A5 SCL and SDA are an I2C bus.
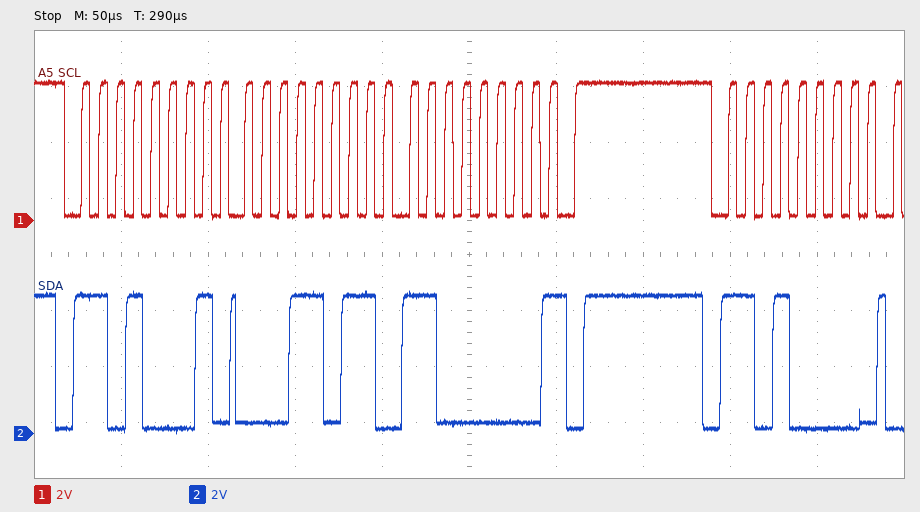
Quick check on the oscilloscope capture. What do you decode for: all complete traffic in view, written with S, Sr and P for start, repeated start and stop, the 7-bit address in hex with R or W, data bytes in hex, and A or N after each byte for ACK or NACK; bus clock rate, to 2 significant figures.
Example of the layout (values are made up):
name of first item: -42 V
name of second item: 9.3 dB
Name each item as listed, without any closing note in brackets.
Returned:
all complete traffic in view, written with S, Sr and P for start, repeated start and stop, the 7-bit address in hex with R or W, data bytes in hex, and A or N after each byte for ACK or NACK: S 68R A 1B A C0 N P S 68W A
bus clock rate, to 2 significant figures: 100 kHz
